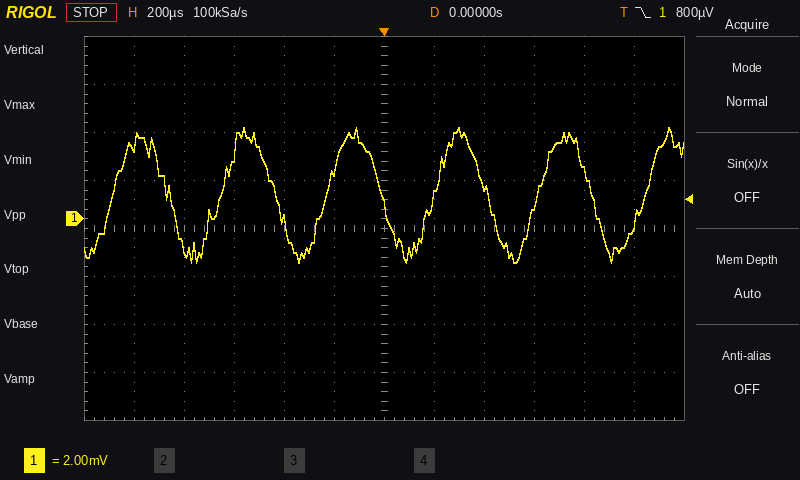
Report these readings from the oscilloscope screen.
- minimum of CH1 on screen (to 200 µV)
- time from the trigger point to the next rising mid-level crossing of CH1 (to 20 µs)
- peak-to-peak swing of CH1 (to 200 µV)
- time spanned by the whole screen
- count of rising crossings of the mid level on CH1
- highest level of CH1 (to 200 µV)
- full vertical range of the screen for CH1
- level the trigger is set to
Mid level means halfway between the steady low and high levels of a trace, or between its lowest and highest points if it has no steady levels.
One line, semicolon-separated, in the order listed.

-1.8 mV; 200 µs; 5.6 mV; 2.4 ms; 6; 3.8 mV; 16 mV; 800 µV
